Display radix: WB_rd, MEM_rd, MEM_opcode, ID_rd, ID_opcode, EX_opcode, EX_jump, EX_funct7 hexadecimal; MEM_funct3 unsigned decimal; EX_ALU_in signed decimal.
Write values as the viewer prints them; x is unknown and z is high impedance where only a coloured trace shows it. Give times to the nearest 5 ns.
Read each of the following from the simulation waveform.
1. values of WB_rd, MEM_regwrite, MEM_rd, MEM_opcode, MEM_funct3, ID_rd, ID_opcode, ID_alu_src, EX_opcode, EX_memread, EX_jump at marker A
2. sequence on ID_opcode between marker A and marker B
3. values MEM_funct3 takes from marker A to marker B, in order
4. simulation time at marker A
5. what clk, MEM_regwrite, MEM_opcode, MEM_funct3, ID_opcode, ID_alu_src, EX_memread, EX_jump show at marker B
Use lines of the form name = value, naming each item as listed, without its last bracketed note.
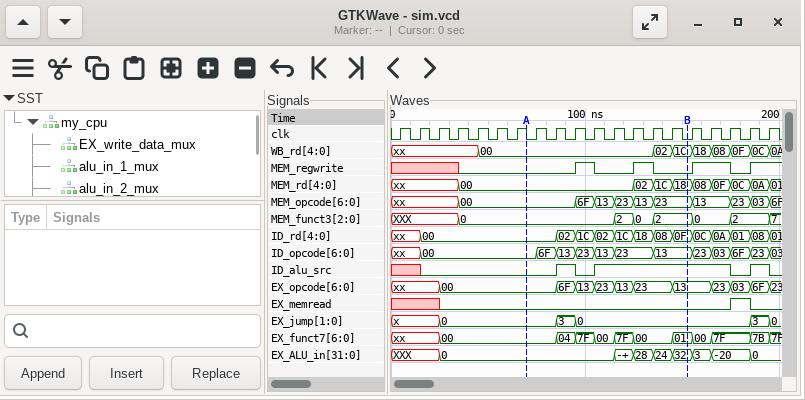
values of WB_rd, MEM_regwrite, MEM_rd, MEM_opcode, MEM_funct3, ID_rd, ID_opcode, ID_alu_src, EX_opcode, EX_memread, EX_jump at marker A = WB_rd=00, MEM_regwrite=0, MEM_rd=00, MEM_opcode=00, MEM_funct3=0, ID_rd=00, ID_opcode=00, ID_alu_src=0, EX_opcode=00, EX_memread=0, EX_jump=0
sequence on ID_opcode between marker A and marker B = 00, 6F, 13, 23, 13, 23, 13
values MEM_funct3 takes from marker A to marker B, in order = 0, 2, 0, 2
simulation time at marker A = 70 ns
what clk, MEM_regwrite, MEM_opcode, MEM_funct3, ID_opcode, ID_alu_src, EX_memread, EX_jump show at marker B = clk=0, MEM_regwrite=0, MEM_opcode=23, MEM_funct3=2, ID_opcode=13, ID_alu_src=1, EX_memread=0, EX_jump=0
